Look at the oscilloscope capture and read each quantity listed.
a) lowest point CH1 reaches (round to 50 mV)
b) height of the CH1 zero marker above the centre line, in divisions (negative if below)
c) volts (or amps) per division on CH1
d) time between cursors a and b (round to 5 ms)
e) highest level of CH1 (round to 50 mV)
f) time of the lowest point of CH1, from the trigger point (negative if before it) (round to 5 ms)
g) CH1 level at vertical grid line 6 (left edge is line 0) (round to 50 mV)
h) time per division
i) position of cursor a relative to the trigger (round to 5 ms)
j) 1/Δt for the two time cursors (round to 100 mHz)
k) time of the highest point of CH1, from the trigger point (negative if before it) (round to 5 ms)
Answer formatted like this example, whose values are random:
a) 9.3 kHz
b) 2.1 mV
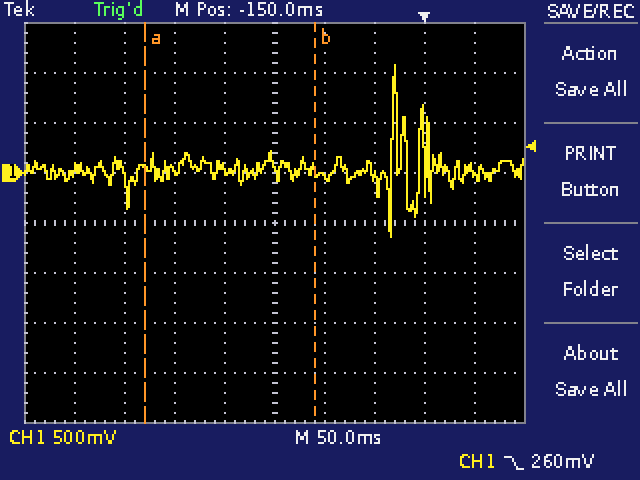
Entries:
a) -650 mV
b) +1.0 div
c) 500 mV
d) 170 ms
e) 1.10 V
f) -35 ms
g) -50 mV
h) 50 ms
i) -280 ms
j) 5.9 Hz
k) -30 ms
